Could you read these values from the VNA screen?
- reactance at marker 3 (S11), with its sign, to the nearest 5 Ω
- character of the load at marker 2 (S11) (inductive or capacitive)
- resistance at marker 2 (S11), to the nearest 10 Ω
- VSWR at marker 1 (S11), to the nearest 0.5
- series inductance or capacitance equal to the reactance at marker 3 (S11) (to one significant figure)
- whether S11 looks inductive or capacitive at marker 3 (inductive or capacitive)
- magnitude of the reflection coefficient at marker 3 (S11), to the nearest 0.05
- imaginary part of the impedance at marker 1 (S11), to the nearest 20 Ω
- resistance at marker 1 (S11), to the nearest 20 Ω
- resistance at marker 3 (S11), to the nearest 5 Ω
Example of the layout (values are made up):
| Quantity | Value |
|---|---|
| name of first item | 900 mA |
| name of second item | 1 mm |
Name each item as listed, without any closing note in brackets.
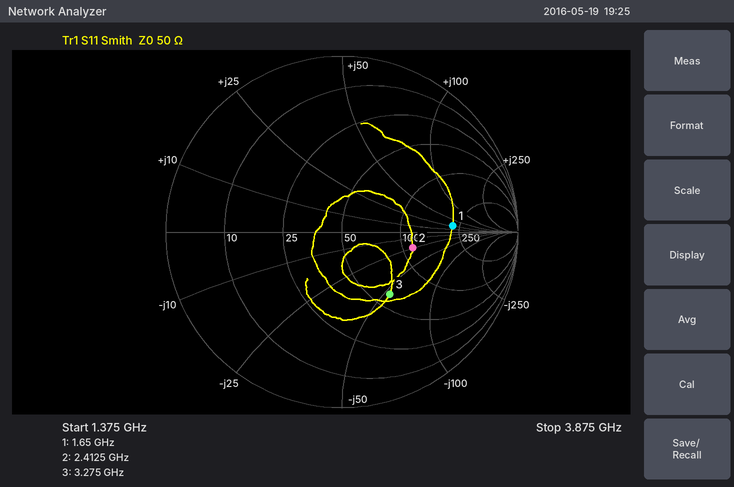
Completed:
| Quantity | Value |
|---|---|
| reactance at marker 3 (S11), with its sign, to the nearest 5 Ω | -55 Ω |
| character of the load at marker 2 (S11) | capacitive |
| resistance at marker 2 (S11), to the nearest 10 Ω | 110 Ω |
| VSWR at marker 1 (S11), to the nearest 0.5 | 4.5 |
| series inductance or capacitance equal to the reactance at marker 3 (S11) | 900 fF |
| whether S11 looks inductive or capacitive at marker 3 | capacitive |
| magnitude of the reflection coefficient at marker 3 (S11), to the nearest 0.05 | 0.45 |
| imaginary part of the impedance at marker 1 (S11), to the nearest 20 Ω | +20 Ω |
| resistance at marker 1 (S11), to the nearest 20 Ω | 220 Ω |
| resistance at marker 3 (S11), to the nearest 5 Ω | 60 Ω |
